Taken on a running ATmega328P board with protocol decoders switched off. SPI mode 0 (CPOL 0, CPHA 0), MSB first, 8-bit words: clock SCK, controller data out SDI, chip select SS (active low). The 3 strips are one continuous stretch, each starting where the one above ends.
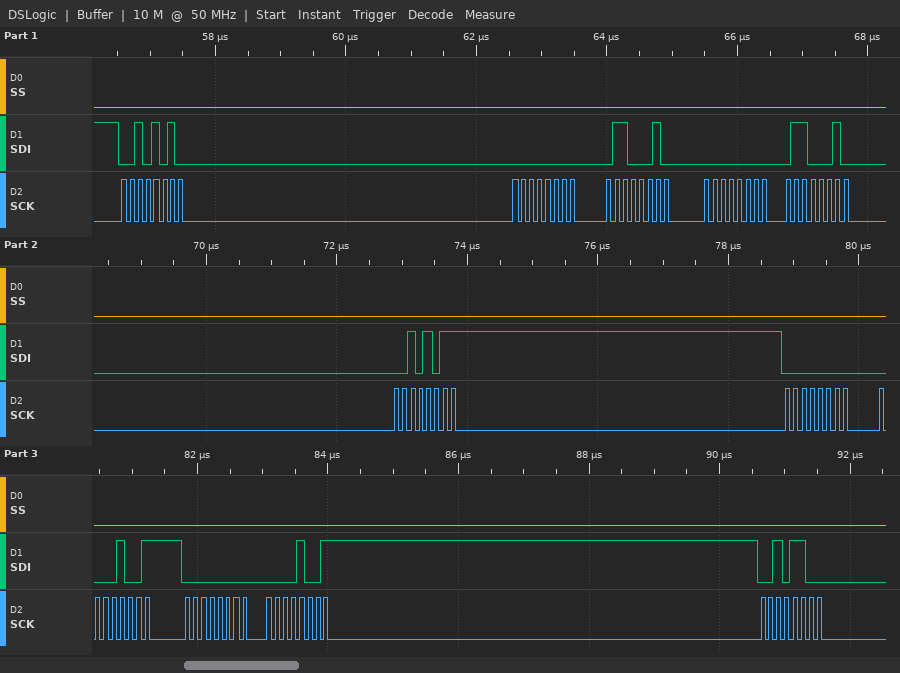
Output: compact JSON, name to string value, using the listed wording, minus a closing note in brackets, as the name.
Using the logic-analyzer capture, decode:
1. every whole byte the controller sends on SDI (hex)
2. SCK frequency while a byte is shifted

{"every whole byte the controller sends on SDI": "2A 00 62 00 62 2B 00 09 00 09 2C", "SCK frequency while a byte is shifted": "8 MHz"}
